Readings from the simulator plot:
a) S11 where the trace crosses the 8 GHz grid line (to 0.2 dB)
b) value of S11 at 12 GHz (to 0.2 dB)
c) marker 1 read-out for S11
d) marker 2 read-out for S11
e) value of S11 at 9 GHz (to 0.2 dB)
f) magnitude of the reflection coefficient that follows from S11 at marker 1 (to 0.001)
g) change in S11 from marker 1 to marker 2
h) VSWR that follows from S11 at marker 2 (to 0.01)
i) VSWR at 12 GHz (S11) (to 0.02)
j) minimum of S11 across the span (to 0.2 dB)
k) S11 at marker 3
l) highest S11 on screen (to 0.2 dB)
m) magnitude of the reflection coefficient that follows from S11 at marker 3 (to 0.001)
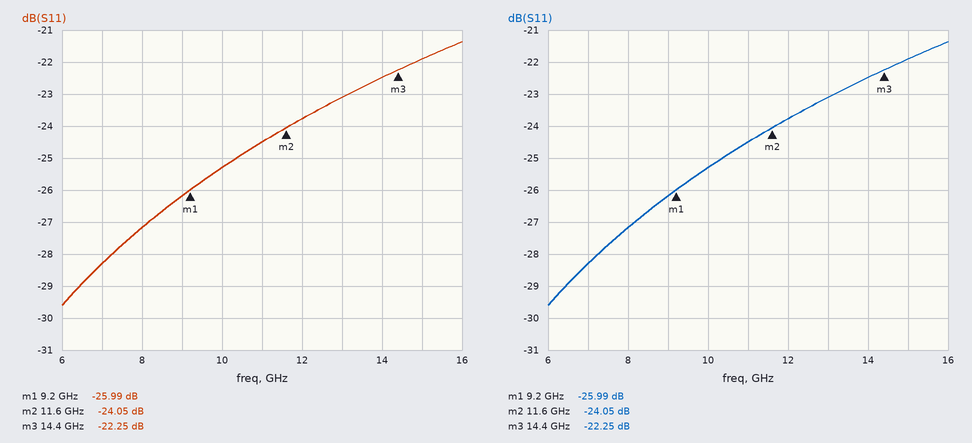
-27.2 dB
-23.8 dB
-25.99 dB
-24.05 dB
-26.2 dB
0.050
1.94 dB
1.13
1.14
-29.6 dB
-22.25 dB
-21.4 dB
0.077
